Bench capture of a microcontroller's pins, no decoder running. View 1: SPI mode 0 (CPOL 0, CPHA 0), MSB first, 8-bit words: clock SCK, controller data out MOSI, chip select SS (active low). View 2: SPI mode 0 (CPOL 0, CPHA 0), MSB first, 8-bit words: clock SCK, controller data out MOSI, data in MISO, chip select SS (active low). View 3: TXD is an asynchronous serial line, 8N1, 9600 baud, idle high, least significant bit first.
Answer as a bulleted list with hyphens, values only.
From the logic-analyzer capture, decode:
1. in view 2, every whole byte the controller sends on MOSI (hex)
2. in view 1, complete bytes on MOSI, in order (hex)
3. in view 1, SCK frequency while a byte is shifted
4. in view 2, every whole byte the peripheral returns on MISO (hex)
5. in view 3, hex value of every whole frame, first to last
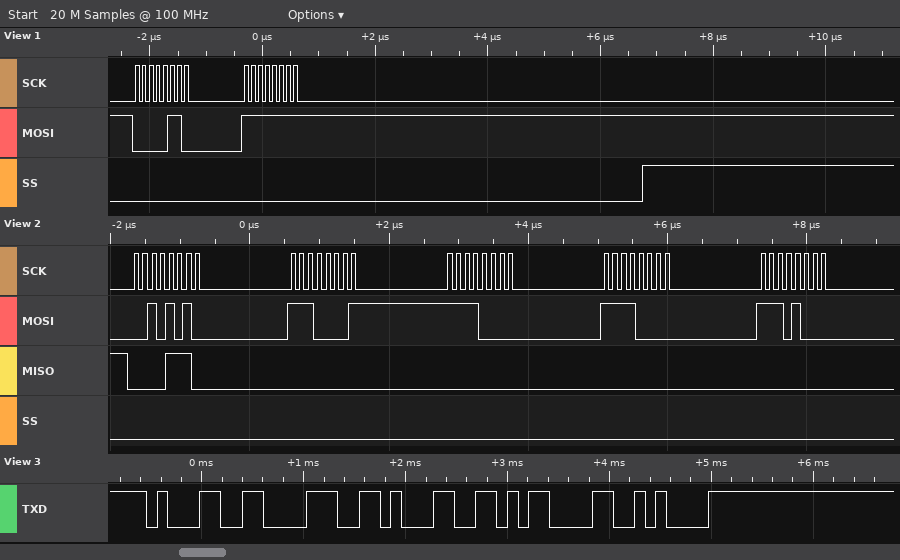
- 2A E1 F0 F0 E8
- 06 FF
- 8 MHz
- 0E 00 00 00 00
- 31 38 31 0D 0A
